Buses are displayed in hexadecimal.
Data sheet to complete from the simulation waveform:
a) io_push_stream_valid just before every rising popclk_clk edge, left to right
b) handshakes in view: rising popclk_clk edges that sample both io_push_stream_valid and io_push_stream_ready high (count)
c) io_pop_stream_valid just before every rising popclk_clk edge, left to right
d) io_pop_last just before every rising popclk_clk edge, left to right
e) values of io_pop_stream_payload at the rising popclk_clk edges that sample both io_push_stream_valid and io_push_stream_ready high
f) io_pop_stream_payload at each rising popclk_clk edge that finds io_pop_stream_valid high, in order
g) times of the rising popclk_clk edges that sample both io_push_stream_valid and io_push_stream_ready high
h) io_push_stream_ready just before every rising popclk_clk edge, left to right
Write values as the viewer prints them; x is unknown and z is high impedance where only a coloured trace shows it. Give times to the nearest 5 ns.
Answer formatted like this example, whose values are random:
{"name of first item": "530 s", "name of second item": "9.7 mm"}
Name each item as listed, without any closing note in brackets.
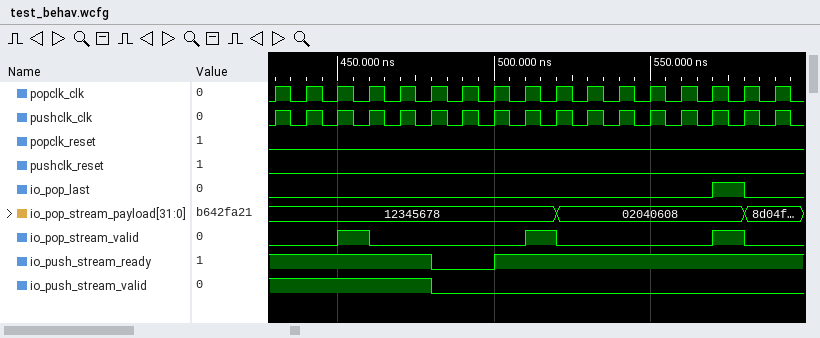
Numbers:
{"io_push_stream_valid just before every rising popclk_clk edge, left to right": "1 1 1 1 1 1 0 0 0 0 0 0 0 0 0 0 0", "handshakes in view: rising popclk_clk edges that sample both io_push_stream_valid and io_push_stream_ready high": "6", "io_pop_stream_valid just before every rising popclk_clk edge, left to right": "0 0 0 1 0 0 0 0 0 1 0 0 0 0 0 1 0", "io_pop_last just before every rising popclk_clk edge, left to right": "0 0 0 0 0 0 0 0 0 0 0 0 0 0 0 1 0", "values of io_pop_stream_payload at the rising popclk_clk edges that sample both io_push_stream_valid and io_push_stream_ready high": "12345678, 12345678, 12345678, 12345678, 12345678, 12345678", "io_pop_stream_payload at each rising popclk_clk edge that finds io_pop_stream_valid high, in order": "12345678, 12345678, 02040608", "times of the rising popclk_clk edges that sample both io_push_stream_valid and io_push_stream_ready high": "430 ns, 440 ns, 450 ns, 460 ns, 470 ns, 480 ns", "io_push_stream_ready just before every rising popclk_clk edge, left to right": "1 1 1 1 1 1 0 0 1 1 1 1 1 1 1 1 1"}
